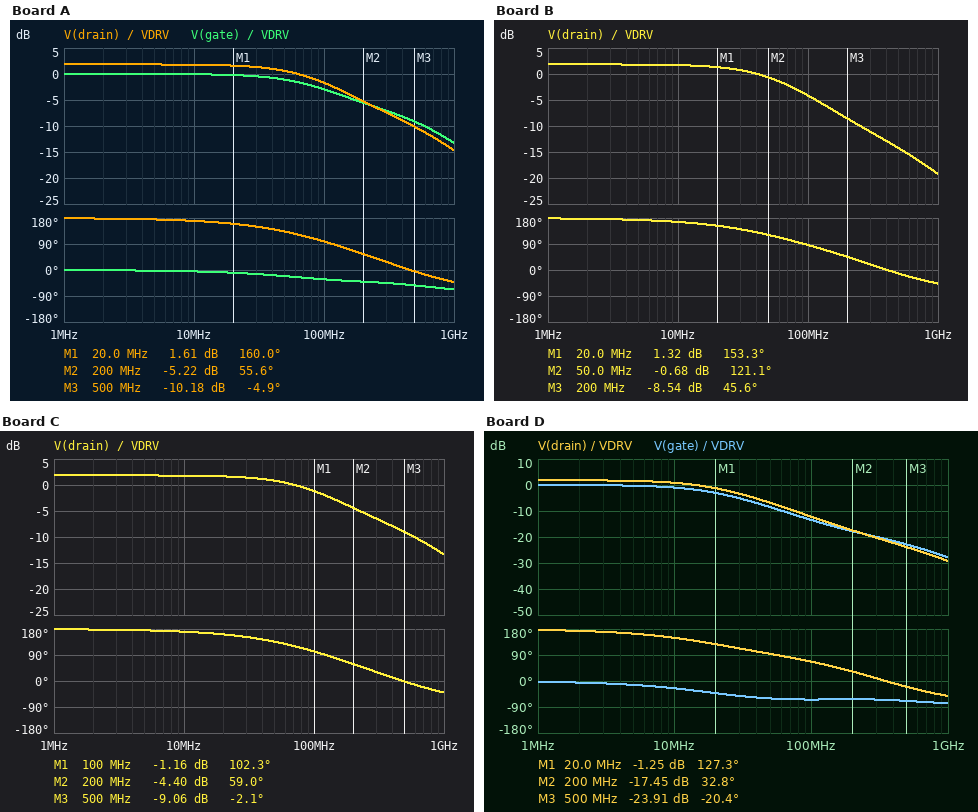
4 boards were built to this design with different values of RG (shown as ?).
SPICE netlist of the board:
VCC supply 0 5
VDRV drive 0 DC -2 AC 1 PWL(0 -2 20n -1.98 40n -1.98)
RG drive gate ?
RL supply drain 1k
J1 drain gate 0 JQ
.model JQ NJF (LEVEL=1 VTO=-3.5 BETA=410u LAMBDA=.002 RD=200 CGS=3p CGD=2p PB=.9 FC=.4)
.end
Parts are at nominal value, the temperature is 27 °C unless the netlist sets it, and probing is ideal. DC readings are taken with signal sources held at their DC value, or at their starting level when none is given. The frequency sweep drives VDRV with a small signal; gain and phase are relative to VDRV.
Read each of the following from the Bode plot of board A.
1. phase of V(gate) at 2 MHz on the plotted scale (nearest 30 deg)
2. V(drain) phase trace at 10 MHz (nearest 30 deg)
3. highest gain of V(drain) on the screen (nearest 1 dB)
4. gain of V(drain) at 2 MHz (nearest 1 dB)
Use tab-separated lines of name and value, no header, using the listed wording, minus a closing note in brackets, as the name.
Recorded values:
phase of V(gate) at 2 MHz on the plotted scale	0 deg
V(drain) phase trace at 10 MHz	180 deg
highest gain of V(drain) on the screen	2 dB
gain of V(drain) at 2 MHz	2 dB
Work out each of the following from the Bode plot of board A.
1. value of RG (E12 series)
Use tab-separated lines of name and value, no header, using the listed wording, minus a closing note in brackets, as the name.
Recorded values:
value of RG	390 Ω
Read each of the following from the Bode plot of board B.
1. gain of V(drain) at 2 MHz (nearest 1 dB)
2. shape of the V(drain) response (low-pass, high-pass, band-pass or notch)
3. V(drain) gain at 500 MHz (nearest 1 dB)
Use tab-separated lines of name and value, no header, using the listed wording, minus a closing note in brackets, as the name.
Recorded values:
gain of V(drain) at 2 MHz	2 dB
shape of the V(drain) response	low-pass
V(drain) gain at 500 MHz	-14 dB
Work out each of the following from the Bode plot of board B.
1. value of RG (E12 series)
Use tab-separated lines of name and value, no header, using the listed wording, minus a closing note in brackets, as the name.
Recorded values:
value of RG	680 Ω
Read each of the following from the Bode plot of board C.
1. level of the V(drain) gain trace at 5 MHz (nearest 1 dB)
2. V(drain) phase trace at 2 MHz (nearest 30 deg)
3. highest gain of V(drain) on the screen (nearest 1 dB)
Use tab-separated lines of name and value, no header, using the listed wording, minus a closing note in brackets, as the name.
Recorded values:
level of the V(drain) gain trace at 5 MHz	2 dB
V(drain) phase trace at 2 MHz	180 deg
highest gain of V(drain) on the screen	2 dB
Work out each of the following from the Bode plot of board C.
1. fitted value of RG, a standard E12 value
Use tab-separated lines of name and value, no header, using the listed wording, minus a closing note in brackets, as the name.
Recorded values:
fitted value of RG, a standard E12 value	330 Ω
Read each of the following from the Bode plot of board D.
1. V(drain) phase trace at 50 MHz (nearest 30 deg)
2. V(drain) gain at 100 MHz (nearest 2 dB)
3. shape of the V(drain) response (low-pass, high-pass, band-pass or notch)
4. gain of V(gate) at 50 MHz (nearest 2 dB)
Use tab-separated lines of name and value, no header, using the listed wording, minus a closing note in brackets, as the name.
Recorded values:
V(drain) phase trace at 50 MHz	90 deg
V(drain) gain at 100 MHz	-12 dB
shape of the V(drain) response	low-pass
gain of V(gate) at 50 MHz	-8 dB
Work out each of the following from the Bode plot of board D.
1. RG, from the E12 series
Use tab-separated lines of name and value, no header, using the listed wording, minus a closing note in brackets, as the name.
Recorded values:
RG, from the E12 series	2.2 kΩ
